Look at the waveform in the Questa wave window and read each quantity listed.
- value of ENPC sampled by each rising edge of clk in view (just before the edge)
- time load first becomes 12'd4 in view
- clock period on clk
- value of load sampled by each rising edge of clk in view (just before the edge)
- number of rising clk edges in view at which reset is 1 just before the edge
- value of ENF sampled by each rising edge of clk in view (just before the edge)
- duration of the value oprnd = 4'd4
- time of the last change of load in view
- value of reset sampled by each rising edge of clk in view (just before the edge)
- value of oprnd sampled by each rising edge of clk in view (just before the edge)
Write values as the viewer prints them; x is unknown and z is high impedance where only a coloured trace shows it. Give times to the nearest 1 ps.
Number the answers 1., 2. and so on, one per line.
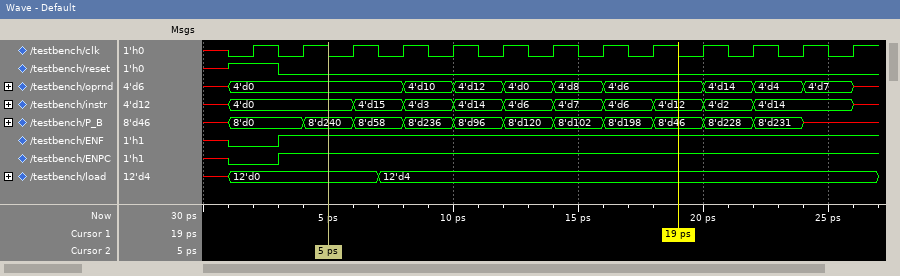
1. 0 1 1 1 1 1 1 1 1 1 1 1 1
2. 7 ps
3. 2 ps
4. 12'd0, 12'd0, 12'd0, 12'd4, 12'd4, 12'd4, 12'd4, 12'd4, 12'd4, 12'd4, 12'd4, 12'd4, 12'd4
5. 1
6. 0 1 1 1 1 1 1 1 1 1 1 1 1
7. 2 ps
8. 7 ps
9. 1 0 0 0 0 0 0 0 0 0 0 0 0
10. 4'd0, 4'd0, 4'd0, 4'd0, 4'd10, 4'd12, 4'd0, 4'd8, 4'd6, 4'd6, 4'd14, 4'd4, 4'd7
